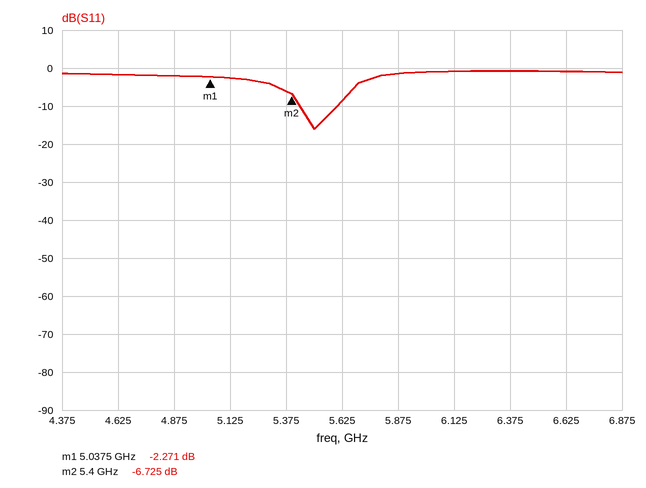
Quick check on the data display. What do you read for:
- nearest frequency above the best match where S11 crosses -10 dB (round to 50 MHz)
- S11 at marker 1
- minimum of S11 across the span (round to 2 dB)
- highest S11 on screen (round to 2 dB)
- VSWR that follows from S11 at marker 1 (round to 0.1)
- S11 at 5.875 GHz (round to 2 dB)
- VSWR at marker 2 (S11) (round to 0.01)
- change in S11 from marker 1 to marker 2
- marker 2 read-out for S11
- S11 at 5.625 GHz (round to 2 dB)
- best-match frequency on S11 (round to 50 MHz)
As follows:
5.60 GHz
-2.271 dB
-16 dB
0 dB
7.7
-2 dB
2.71
-4.454 dB
-6.725 dB
-8 dB
5.50 GHz
